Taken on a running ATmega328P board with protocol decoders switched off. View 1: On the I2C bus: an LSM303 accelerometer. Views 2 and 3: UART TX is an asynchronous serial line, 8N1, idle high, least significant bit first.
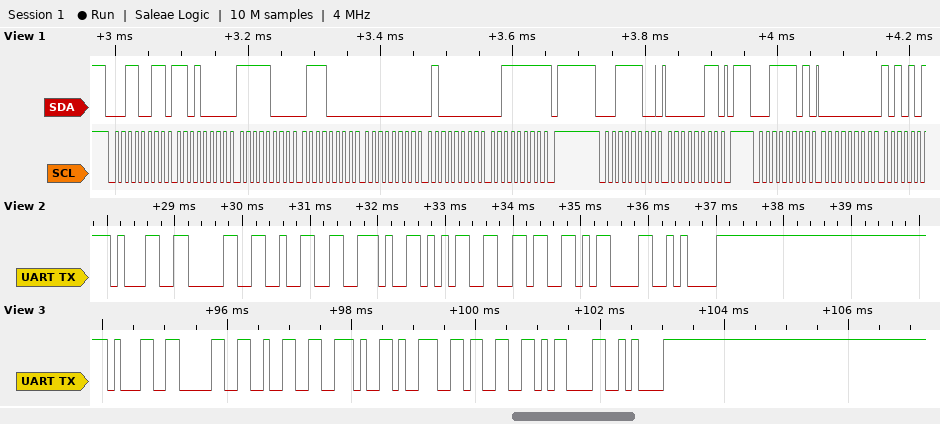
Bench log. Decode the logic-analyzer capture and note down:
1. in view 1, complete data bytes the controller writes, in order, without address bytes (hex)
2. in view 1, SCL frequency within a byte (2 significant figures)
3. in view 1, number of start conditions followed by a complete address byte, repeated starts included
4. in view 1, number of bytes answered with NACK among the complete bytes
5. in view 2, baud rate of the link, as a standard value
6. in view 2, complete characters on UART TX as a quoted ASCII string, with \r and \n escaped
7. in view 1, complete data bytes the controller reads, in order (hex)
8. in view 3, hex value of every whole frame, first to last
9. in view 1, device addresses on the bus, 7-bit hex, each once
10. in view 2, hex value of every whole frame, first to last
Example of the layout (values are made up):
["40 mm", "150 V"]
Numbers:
["03", "100 kHz", "3", "1", "9600 baud", "\"102.56\\r\\n\"", "D0 F8 70 00 40 3F 00", "31 30 32 2E 39 33 0D 0A", "0x19 0x1E", "0x31 0x30 0x32 0x2E 0x35 0x36 0x0D 0x0A"]
